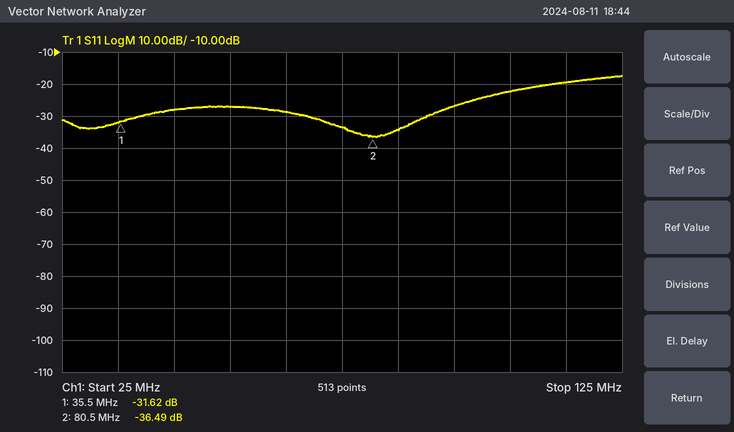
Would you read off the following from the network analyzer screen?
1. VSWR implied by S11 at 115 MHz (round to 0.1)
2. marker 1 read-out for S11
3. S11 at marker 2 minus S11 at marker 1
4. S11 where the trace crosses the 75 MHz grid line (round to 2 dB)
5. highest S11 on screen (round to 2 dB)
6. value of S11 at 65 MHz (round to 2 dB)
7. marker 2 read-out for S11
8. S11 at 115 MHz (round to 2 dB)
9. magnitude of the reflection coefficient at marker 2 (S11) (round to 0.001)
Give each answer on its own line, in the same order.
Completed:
1.2
-31.62 dB
-4.87 dB
-34 dB
-18 dB
-28 dB
-36.49 dB
-20 dB
0.015
